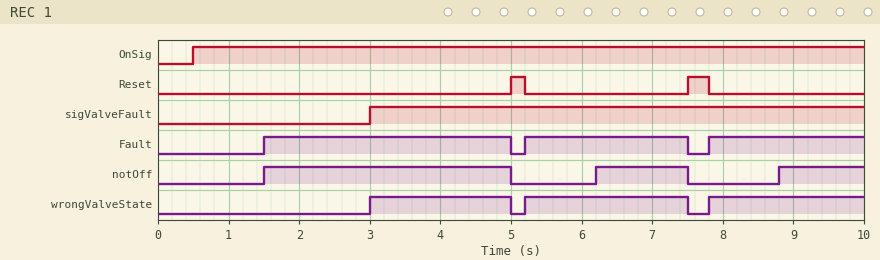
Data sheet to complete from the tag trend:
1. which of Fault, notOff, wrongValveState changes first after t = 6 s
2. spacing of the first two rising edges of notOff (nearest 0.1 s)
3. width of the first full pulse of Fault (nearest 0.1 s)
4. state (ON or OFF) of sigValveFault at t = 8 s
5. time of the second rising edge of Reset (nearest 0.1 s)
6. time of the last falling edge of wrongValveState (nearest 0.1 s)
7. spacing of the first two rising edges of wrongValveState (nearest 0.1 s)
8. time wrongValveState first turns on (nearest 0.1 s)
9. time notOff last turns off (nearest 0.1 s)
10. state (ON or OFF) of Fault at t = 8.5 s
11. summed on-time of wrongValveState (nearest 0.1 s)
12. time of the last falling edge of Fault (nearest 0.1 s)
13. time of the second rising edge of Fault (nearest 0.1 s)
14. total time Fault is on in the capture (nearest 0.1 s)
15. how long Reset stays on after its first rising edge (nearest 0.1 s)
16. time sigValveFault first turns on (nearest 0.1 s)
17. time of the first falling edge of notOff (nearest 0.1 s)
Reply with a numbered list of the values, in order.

1. notOff
2. 4.7 s
3. 3.5 s
4. ON
5. 7.5 s
6. 7.5 s
7. 2.2 s
8. 3.0 s
9. 7.5 s
10. ON
11. 6.5 s
12. 7.5 s
13. 5.2 s
14. 8.0 s
15. 0.2 s
16. 3.0 s
17. 5.0 s
